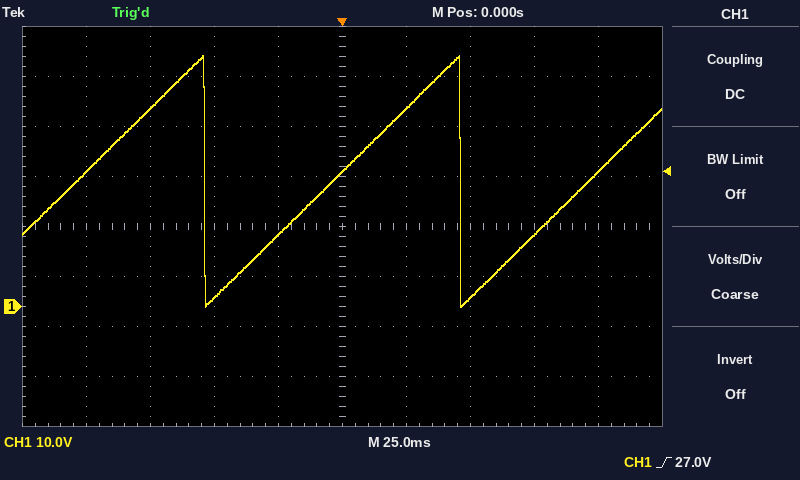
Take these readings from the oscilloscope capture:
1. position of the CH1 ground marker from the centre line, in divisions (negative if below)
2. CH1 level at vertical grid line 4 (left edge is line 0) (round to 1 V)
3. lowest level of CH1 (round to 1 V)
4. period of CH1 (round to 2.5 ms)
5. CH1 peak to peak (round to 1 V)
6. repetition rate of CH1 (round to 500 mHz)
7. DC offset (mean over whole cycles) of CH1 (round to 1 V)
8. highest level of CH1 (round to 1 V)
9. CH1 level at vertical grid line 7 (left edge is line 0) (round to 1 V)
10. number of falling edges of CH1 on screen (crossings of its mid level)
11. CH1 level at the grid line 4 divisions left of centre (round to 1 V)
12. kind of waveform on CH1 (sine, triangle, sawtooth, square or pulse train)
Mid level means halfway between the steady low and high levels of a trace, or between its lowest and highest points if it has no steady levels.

-1.6 div
14 V
0 V
100.0 ms
50 V
10.0 Hz
25 V
50 V
2 V
2
27 V
sawtooth
